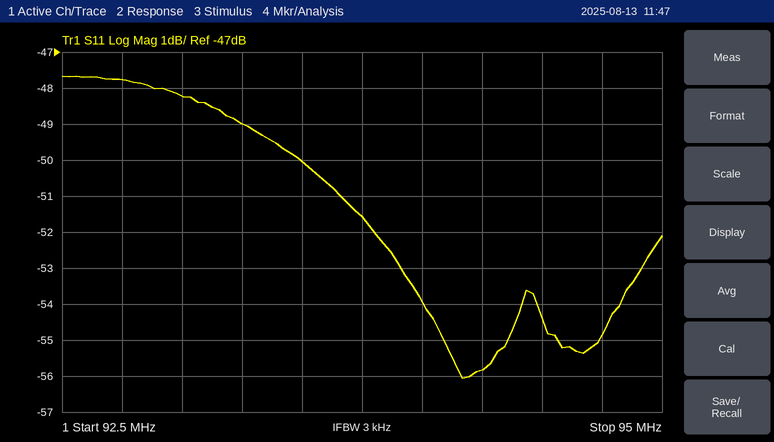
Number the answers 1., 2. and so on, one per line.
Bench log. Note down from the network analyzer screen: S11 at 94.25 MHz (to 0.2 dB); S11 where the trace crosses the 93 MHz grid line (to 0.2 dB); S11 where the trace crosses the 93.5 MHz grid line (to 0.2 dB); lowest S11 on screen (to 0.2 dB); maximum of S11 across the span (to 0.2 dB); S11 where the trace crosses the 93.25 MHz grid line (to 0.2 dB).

1. -55.8 dB
2. -48.2 dB
3. -50.0 dB
4. -56.0 dB
5. -47.6 dB
6. -49.0 dB
